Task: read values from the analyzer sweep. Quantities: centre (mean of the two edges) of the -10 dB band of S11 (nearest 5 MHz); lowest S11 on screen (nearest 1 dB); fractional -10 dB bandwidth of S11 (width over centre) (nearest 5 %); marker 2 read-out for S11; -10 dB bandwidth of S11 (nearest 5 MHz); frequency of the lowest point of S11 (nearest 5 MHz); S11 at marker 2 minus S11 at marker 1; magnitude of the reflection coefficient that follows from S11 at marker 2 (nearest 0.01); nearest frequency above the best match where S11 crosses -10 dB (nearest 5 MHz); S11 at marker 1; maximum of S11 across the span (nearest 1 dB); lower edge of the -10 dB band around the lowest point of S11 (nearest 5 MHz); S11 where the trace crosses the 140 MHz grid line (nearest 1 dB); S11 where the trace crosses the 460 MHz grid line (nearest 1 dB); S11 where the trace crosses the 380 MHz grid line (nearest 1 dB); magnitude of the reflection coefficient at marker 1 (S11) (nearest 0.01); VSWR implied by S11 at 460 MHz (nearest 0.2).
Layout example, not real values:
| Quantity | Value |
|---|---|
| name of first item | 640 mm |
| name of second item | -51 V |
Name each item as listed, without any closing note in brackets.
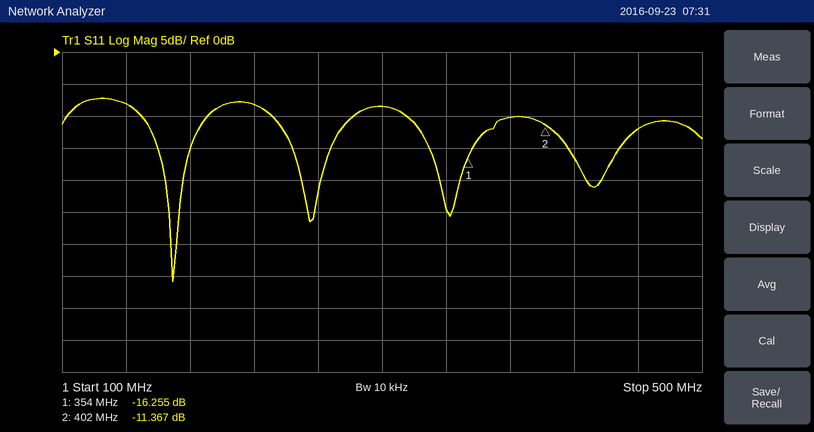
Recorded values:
| Quantity | Value |
|---|---|
| centre (mean of the two edges) of the -10 dB band of S11 | 170 MHz |
| lowest S11 on screen | -36 dB |
| fractional -10 dB bandwidth of S11 (width over centre) | 25 % |
| marker 2 read-out for S11 | -11.367 dB |
| -10 dB bandwidth of S11 | 40 MHz |
| frequency of the lowest point of S11 | 170 MHz |
| S11 at marker 2 minus S11 at marker 1 | 4.888 dB |
| magnitude of the reflection coefficient that follows from S11 at marker 2 | 0.27 |
| nearest frequency above the best match where S11 crosses -10 dB | 190 MHz |
| S11 at marker 1 | -16.255 dB |
| maximum of S11 across the span | -7 dB |
| lower edge of the -10 dB band around the lowest point of S11 | 150 MHz |
| S11 where the trace crosses the 140 MHz grid line | -8 dB |
| S11 where the trace crosses the 460 MHz grid line | -12 dB |
| S11 where the trace crosses the 380 MHz grid line | -10 dB |
| magnitude of the reflection coefficient at marker 1 (S11) | 0.15 |
| VSWR implied by S11 at 460 MHz | 1.6 |
